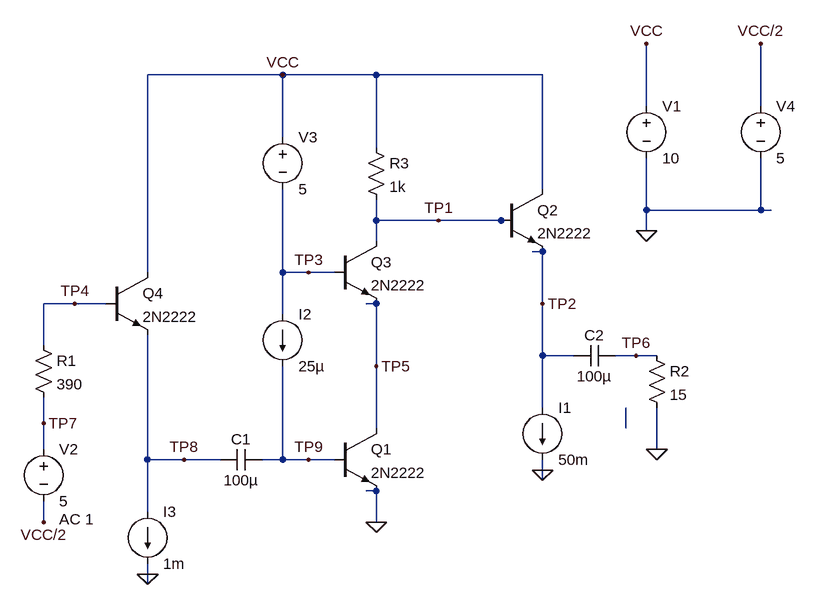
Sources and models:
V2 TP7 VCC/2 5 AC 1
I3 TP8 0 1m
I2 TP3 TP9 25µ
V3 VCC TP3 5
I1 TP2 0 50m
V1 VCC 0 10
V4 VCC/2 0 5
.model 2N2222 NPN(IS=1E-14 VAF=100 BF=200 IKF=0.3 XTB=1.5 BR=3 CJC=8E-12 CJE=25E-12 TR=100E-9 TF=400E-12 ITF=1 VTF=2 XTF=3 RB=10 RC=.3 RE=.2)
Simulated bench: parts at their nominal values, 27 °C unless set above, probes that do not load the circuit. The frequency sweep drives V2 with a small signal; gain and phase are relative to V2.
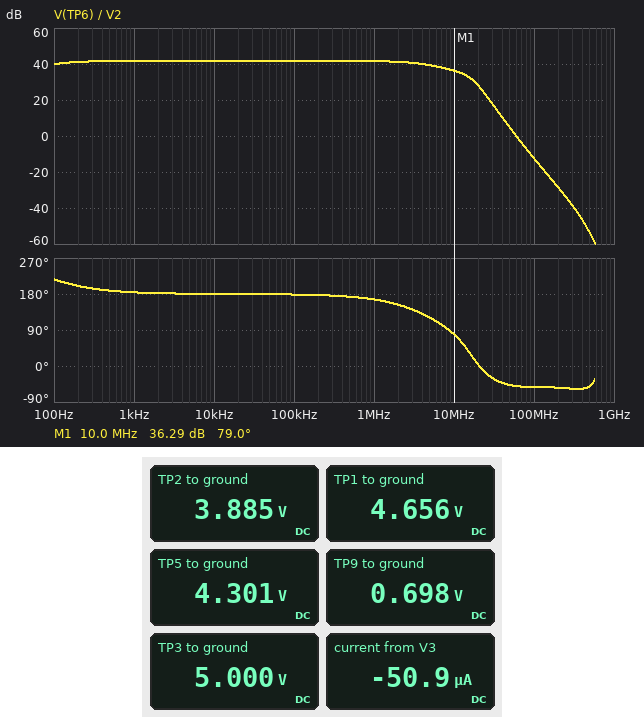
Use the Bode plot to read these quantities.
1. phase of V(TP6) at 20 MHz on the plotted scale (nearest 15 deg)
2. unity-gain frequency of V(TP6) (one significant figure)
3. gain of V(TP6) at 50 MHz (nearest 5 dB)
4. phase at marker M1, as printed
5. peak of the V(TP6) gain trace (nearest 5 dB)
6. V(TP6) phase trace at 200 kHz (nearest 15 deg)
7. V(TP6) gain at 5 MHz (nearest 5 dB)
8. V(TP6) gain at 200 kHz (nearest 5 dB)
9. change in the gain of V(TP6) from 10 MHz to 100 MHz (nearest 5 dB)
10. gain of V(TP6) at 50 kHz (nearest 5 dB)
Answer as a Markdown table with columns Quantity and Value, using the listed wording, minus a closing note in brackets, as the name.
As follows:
| Quantity | Value |
|---|---|
| phase of V(TP6) at 20 MHz on the plotted scale | 0 deg |
| unity-gain frequency of V(TP6) | 60 MHz |
| gain of V(TP6) at 50 MHz | 5 dB |
| phase at marker M1, as printed | 79.0 deg |
| peak of the V(TP6) gain trace | 40 dB |
| V(TP6) phase trace at 200 kHz | 180 deg |
| V(TP6) gain at 5 MHz | 40 dB |
| V(TP6) gain at 200 kHz | 40 dB |
| change in the gain of V(TP6) from 10 MHz to 100 MHz | -50 dB |
| gain of V(TP6) at 50 kHz | 40 dB |
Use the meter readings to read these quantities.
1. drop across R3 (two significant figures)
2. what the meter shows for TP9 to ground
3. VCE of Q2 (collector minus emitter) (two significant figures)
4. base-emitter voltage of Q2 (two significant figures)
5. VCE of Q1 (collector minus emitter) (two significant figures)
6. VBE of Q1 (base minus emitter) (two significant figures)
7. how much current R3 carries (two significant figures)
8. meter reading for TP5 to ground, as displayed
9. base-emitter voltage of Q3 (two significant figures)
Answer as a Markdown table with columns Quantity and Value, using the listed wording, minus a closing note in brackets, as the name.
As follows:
| Quantity | Value |
|---|---|
| drop across R3 | 5.3 V |
| what the meter shows for TP9 to ground | 0.698 V |
| VCE of Q2 (collector minus emitter) | 6.1 V |
| base-emitter voltage of Q2 | 770 mV |
| VCE of Q1 (collector minus emitter) | 4.3 V |
| VBE of Q1 (base minus emitter) | 700 mV |
| how much current R3 carries | 5.3 mA |
| meter reading for TP5 to ground, as displayed | 4.301 V |
| base-emitter voltage of Q3 | 700 mV |
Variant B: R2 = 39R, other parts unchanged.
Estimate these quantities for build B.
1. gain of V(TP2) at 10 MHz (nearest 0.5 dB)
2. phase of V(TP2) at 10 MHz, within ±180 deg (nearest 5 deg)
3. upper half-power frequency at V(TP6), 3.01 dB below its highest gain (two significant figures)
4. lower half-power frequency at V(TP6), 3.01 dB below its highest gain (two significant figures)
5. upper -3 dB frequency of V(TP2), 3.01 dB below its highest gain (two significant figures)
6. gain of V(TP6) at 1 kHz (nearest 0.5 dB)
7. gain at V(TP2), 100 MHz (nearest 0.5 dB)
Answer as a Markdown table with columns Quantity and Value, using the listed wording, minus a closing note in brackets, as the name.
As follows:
| Quantity | Value |
|---|---|
| gain of V(TP2) at 10 MHz | 40.0 dB |
| phase of V(TP2) at 10 MHz, within ±180 deg | 85 deg |
| upper half-power frequency at V(TP6), 3.01 dB below its highest gain | 9.1 MHz |
| lower half-power frequency at V(TP6), 3.01 dB below its highest gain | 35 Hz |
| upper -3 dB frequency of V(TP2), 3.01 dB below its highest gain | 6.2 MHz |
| gain of V(TP6) at 1 kHz | 43.5 dB |
| gain at V(TP2), 100 MHz | -8.0 dB |
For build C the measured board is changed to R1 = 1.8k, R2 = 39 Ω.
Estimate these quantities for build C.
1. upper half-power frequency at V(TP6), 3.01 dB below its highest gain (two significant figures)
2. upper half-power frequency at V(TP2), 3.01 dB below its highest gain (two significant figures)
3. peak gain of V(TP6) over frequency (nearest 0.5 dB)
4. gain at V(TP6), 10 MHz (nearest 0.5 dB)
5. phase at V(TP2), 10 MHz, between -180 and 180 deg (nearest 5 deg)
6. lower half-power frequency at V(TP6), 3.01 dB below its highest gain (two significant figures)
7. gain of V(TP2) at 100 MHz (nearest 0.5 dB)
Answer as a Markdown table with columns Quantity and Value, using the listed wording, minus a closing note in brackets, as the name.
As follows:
| Quantity | Value |
|---|---|
| upper half-power frequency at V(TP6), 3.01 dB below its highest gain | 6.9 MHz |
| upper half-power frequency at V(TP2), 3.01 dB below its highest gain | 5.7 MHz |
| peak gain of V(TP6) over frequency | 43.5 dB |
| gain at V(TP6), 10 MHz | 35.5 dB |
| phase at V(TP2), 10 MHz, between -180 and 180 deg | 20 deg |
| lower half-power frequency at V(TP6), 3.01 dB below its highest gain | 35 Hz |
| gain of V(TP2) at 100 MHz | -21.0 dB |
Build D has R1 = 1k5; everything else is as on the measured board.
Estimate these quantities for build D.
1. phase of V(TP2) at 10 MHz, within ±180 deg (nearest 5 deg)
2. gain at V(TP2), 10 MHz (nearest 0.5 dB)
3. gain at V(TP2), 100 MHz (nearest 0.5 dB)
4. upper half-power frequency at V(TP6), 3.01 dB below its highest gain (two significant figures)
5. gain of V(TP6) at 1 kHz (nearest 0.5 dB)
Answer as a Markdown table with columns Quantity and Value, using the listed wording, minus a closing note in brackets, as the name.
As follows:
| Quantity | Value |
|---|---|
| phase of V(TP2) at 10 MHz, within ±180 deg | 20 deg |
| gain at V(TP2), 10 MHz | 33.0 dB |
| gain at V(TP2), 100 MHz | -24.0 dB |
| upper half-power frequency at V(TP6), 3.01 dB below its highest gain | 6.1 MHz |
| gain of V(TP6) at 1 kHz | 41.5 dB |
